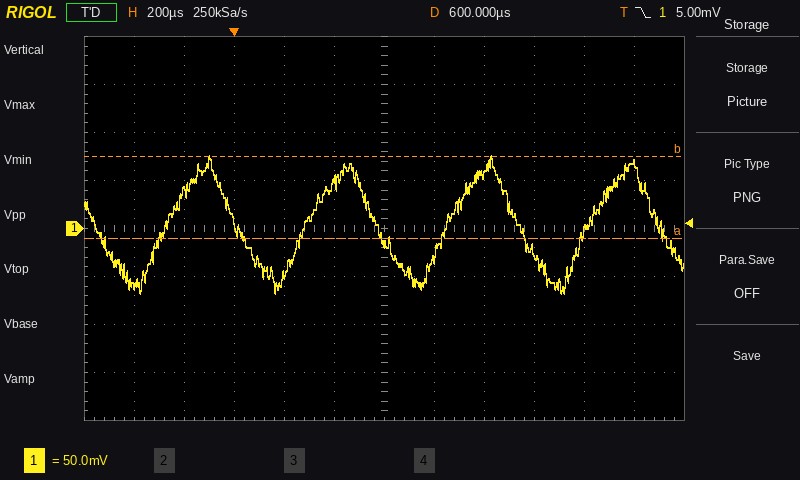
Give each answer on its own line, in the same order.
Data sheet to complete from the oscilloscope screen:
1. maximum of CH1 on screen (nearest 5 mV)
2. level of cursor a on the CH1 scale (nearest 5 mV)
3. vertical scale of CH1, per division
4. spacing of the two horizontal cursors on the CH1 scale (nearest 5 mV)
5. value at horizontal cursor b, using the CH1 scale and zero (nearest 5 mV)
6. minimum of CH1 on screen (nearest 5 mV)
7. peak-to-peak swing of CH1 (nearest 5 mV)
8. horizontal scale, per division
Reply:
75 mV
-10 mV
50 mV
85 mV
75 mV
-70 mV
145 mV
200 µs
